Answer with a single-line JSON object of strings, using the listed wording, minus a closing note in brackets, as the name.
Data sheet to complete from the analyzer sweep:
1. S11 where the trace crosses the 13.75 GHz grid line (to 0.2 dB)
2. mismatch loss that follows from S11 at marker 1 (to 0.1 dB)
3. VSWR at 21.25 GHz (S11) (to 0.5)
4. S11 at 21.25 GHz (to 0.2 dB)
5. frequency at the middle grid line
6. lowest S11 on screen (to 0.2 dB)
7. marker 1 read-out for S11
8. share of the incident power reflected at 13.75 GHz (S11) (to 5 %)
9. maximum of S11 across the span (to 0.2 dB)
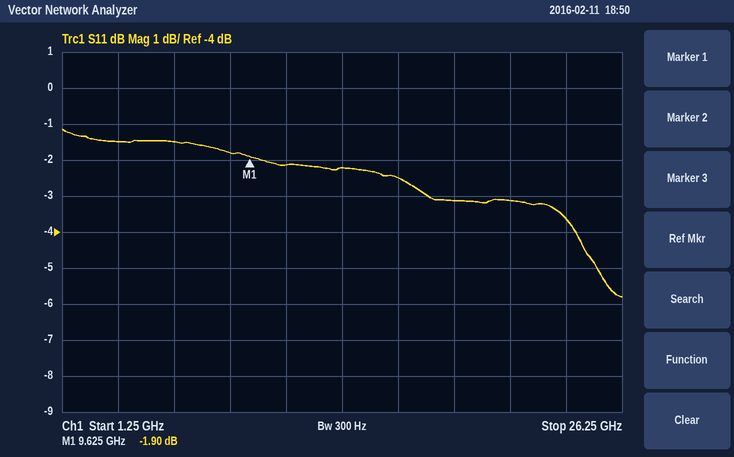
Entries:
{"S11 where the trace crosses the 13.75 GHz grid line": "-2.2 dB", "mismatch loss that follows from S11 at marker 1": "4.5 dB", "VSWR at 21.25 GHz (S11)": "5.5", "S11 at 21.25 GHz": "-3.2 dB", "frequency at the middle grid line": "13.75 GHz", "lowest S11 on screen": "-5.8 dB", "marker 1 read-out for S11": "-1.90 dB", "share of the incident power reflected at 13.75 GHz (S11)": "60 %", "maximum of S11 across the span": "-1.2 dB"}
